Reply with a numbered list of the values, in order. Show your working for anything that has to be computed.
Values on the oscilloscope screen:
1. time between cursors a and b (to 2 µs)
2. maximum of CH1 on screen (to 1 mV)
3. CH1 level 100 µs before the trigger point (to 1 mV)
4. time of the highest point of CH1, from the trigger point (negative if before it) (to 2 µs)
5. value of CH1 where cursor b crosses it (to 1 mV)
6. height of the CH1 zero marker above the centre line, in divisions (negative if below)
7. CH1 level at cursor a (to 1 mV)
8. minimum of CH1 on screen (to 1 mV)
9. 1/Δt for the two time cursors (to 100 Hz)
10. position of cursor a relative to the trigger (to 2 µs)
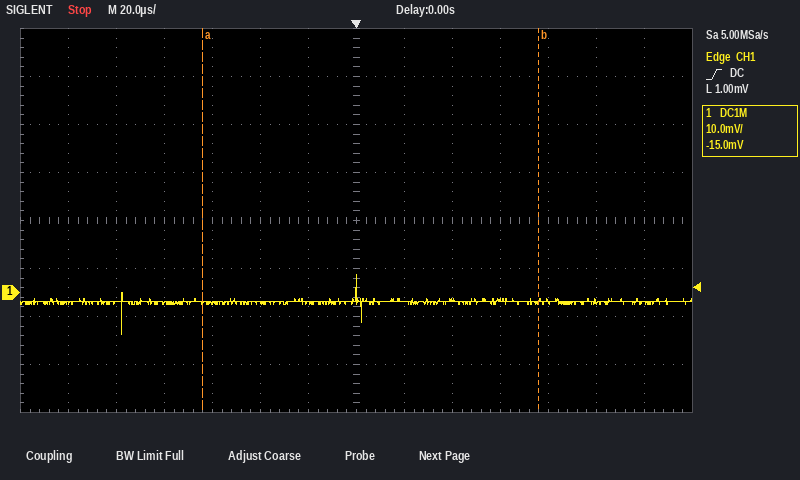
1. 140 µs
2. 4 mV
3. -2 mV
4. 0 µs
5. -2 mV
6. -1.5 div
7. -2 mV
8. -9 mV
9. 1 / 140 µs ≈ 7.1 kHz
10. -64 µs
